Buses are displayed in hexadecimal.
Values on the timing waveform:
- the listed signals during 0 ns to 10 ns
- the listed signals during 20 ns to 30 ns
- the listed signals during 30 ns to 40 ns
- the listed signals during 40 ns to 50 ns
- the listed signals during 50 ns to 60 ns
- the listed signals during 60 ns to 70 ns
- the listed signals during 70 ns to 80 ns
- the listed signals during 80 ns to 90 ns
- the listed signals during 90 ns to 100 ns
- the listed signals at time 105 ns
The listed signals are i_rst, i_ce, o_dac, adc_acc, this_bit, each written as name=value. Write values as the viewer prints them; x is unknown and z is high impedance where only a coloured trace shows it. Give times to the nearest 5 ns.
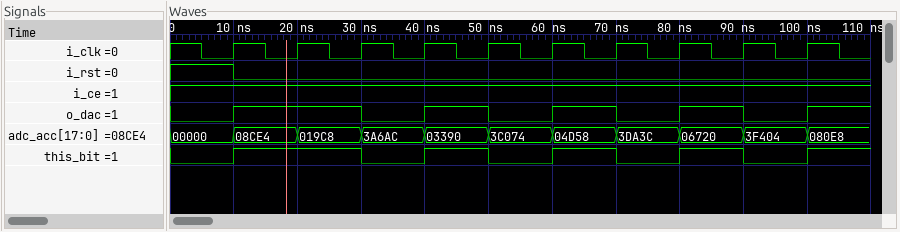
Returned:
i_rst=1, i_ce=1, o_dac=0, adc_acc=00000, this_bit=0
i_rst=0, i_ce=1, o_dac=1, adc_acc=019C8, this_bit=1
i_rst=0, i_ce=1, o_dac=0, adc_acc=3A6AC, this_bit=0
i_rst=0, i_ce=1, o_dac=1, adc_acc=03390, this_bit=1
i_rst=0, i_ce=1, o_dac=0, adc_acc=3C074, this_bit=0
i_rst=0, i_ce=1, o_dac=1, adc_acc=04D58, this_bit=1
i_rst=0, i_ce=1, o_dac=0, adc_acc=3DA3C, this_bit=0
i_rst=0, i_ce=1, o_dac=1, adc_acc=06720, this_bit=1
i_rst=0, i_ce=1, o_dac=0, adc_acc=3F404, this_bit=0
i_rst=0, i_ce=1, o_dac=1, adc_acc=080E8, this_bit=1
